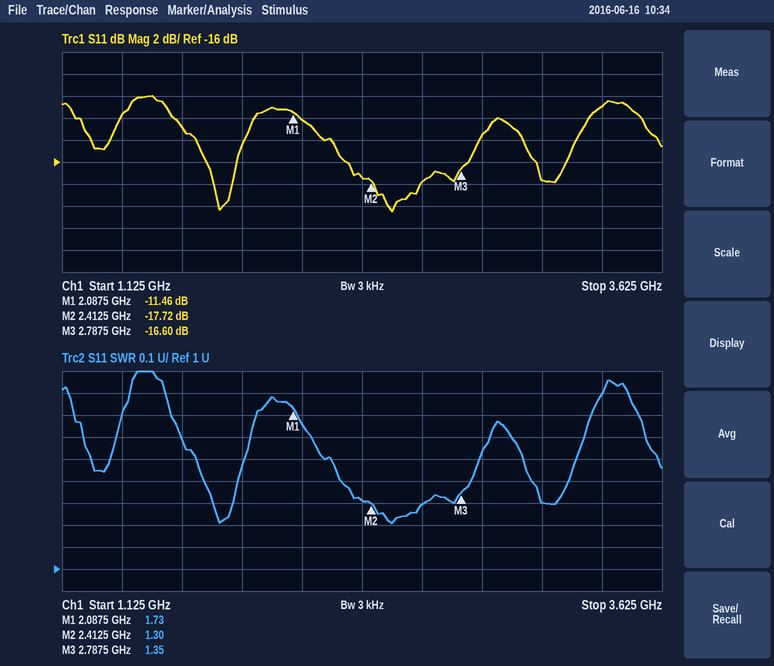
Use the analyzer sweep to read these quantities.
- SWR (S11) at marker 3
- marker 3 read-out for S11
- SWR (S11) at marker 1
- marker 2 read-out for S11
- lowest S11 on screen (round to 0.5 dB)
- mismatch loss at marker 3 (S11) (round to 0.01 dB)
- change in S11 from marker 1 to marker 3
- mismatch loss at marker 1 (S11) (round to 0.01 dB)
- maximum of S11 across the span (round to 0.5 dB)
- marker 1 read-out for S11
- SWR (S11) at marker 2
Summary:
1.35
-16.60 dB
1.73
-17.72 dB
-20.5 dB
0.10 dB
-5.14 dB
0.32 dB
-10.0 dB
-11.46 dB
1.30
